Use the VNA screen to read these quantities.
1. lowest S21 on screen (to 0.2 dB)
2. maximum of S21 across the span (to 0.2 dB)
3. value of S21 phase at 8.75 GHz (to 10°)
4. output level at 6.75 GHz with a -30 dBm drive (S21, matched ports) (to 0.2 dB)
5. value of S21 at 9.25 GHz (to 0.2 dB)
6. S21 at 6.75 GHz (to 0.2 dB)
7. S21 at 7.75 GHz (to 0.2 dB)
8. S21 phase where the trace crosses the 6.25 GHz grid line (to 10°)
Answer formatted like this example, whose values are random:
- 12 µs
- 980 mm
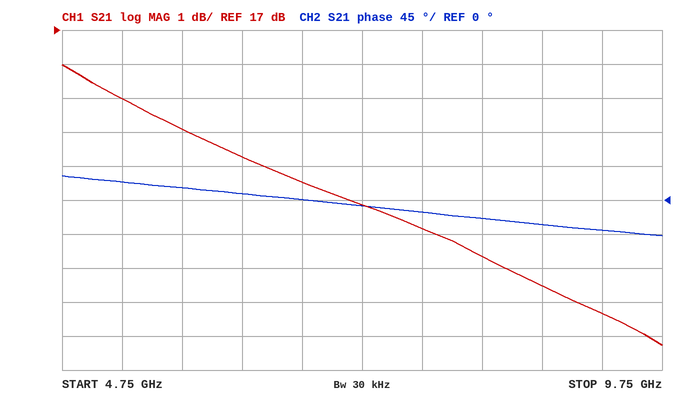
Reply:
- 7.8 dB
- 16.0 dB
- -30°
- -17.4 dBm
- 8.6 dB
- 12.6 dB
- 11.2 dB
- 10°
